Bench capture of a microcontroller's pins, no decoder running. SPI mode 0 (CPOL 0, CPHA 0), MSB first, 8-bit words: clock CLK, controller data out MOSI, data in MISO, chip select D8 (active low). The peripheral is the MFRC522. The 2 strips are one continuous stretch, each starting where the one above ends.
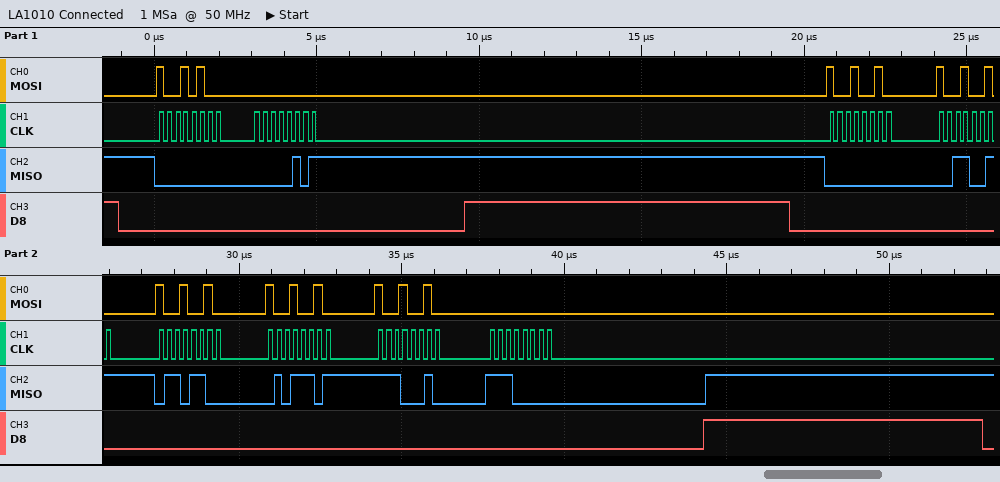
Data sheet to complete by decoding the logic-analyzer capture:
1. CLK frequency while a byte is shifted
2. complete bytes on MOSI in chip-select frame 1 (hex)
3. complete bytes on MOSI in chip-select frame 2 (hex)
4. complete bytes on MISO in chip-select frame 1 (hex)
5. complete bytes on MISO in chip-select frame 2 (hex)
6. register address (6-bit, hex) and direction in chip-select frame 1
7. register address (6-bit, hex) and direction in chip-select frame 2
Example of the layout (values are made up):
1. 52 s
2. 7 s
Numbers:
1. 4 MHz
2. 94 00
3. 92 92 92 92 92 00
4. 00 05
5. 00 33 6C 5D E2 E0
6. 0x0A read
7. 0x09 read
